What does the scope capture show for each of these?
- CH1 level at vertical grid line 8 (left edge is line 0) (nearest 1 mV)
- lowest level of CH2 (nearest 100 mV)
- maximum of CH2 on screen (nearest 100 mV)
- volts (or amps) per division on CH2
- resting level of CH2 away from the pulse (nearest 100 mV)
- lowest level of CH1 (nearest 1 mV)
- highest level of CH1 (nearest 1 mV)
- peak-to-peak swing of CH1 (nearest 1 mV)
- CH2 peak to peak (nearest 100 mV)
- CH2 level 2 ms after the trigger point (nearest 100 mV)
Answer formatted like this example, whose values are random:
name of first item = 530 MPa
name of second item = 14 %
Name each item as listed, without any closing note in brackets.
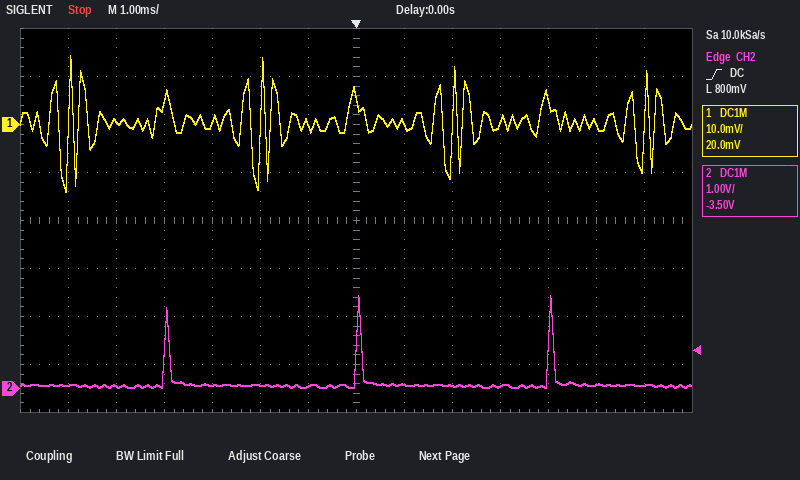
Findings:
CH1 level at vertical grid line 8 (left edge is line 0) = 0 mV
lowest level of CH2 = 0.0 V
maximum of CH2 on screen = 1.9 V
volts (or amps) per division on CH2 = 1 V
resting level of CH2 away from the pulse = 100 mV
lowest level of CH1 = -14 mV
highest level of CH1 = 14 mV
peak-to-peak swing of CH1 = 28 mV
CH2 peak to peak = 1.9 V
CH2 level 2 ms after the trigger point = 100 mV
